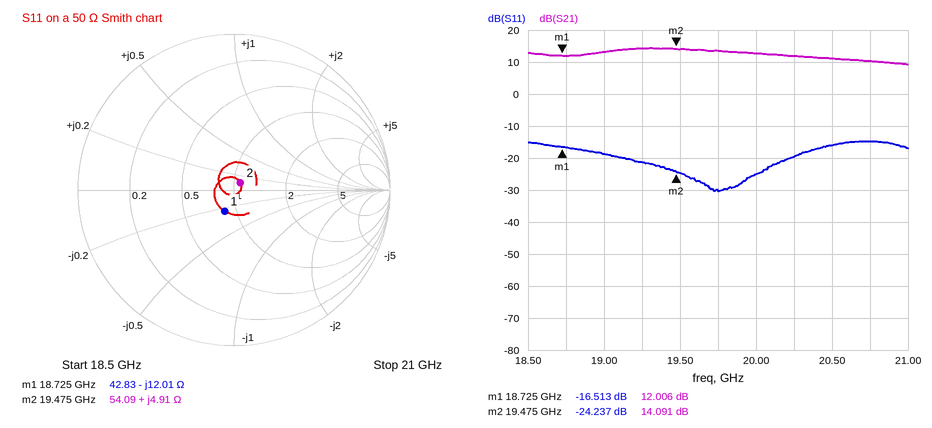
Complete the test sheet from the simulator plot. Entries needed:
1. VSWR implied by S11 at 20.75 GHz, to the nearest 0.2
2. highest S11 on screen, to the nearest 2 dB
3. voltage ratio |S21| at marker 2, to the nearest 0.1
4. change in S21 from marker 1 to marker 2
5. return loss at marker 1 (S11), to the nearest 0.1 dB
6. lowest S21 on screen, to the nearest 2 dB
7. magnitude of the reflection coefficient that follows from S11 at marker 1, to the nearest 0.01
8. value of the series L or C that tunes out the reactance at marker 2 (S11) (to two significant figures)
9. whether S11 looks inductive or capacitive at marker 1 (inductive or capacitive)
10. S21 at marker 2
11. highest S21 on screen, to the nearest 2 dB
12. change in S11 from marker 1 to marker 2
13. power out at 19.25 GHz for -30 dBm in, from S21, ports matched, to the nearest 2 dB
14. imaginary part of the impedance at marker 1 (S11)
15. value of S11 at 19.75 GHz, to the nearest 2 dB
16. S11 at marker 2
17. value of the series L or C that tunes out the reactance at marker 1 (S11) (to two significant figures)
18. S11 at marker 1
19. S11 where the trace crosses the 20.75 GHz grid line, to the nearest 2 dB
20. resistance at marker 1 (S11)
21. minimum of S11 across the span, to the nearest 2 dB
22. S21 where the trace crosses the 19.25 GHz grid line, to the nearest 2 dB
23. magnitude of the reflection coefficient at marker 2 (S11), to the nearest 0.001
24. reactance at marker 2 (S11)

1.4
-14 dB
5.1
2.085 dB
16.5 dB
10 dB
0.15
1.7 pF
capacitive
14.091 dB
14 dB
-7.724 dB
-16 dBm
-12.01 Ω
-30 dB
-24.237 dB
100 pH
-16.513 dB
-14 dB
42.83 Ω
-30 dB
14 dB
0.061
+4.91 Ω
